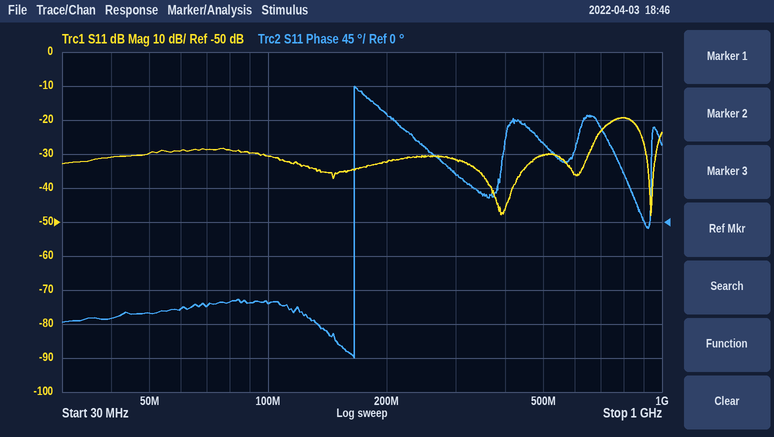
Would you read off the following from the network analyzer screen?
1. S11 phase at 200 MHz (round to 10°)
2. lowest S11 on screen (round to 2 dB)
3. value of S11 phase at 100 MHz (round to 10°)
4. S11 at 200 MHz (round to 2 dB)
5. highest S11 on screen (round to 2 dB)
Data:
140°
-48 dB
-110°
-32 dB
-20 dB
